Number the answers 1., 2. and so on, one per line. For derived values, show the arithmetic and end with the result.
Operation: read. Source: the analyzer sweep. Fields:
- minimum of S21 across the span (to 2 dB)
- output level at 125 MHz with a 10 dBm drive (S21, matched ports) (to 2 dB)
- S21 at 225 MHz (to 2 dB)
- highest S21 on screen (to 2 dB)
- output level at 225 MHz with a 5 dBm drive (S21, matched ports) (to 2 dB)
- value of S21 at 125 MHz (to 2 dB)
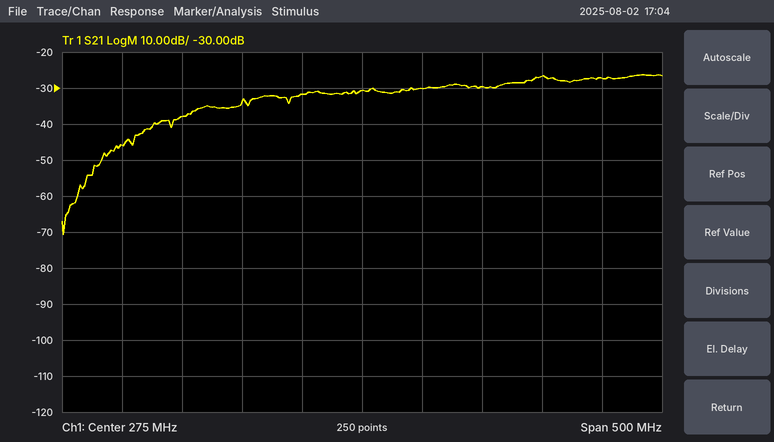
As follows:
1. -70 dB
2. 10 dBm + (-38 dB) = -28 dBm
3. -32 dB
4. -26 dB
5. 5 dBm + (-32 dB) = -26 dBm
6. -38 dB
